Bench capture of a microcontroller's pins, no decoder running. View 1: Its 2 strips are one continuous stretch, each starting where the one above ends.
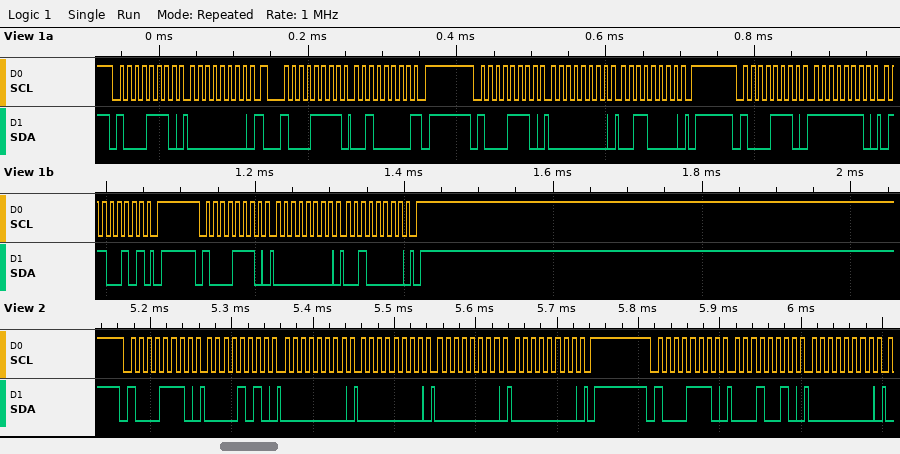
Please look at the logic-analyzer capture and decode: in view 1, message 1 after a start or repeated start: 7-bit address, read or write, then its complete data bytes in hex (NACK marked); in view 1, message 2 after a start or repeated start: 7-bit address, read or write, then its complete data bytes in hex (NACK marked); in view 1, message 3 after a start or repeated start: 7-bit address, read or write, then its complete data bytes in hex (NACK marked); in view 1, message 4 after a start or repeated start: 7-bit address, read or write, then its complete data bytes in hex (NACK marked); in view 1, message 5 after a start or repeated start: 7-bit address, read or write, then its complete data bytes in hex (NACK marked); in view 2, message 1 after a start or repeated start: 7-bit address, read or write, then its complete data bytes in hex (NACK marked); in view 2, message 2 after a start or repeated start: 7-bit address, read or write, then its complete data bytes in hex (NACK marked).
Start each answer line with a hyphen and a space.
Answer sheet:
- 0x47 write: 00
- 0x47 read: 20 NACK
- 0x47 write: 00 30
- 0x47 write: FE 65
- 0x47 write: 00 20
- 0x47 write: 0A 00 00 00 00
- 0x47 write: 12 00
